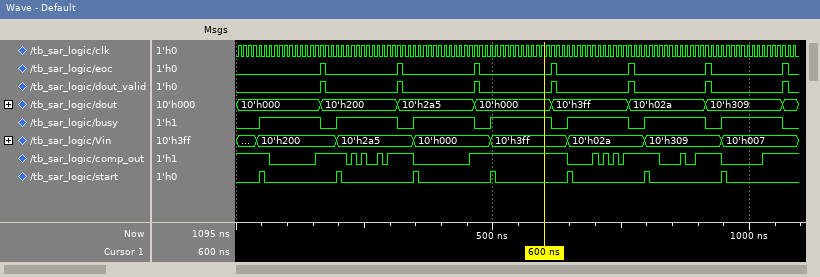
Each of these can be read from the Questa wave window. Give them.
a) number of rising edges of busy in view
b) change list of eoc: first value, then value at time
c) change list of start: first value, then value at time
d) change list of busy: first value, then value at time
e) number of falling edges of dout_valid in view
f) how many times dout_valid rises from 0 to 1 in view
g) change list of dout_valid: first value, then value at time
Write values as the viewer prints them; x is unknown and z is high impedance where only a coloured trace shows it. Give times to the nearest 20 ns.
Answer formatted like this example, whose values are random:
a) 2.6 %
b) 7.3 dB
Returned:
a) 7
b) 0, 1 at 160 ns, 0 at 180 ns, 1 at 320 ns, 0 at 320 ns, 1 at 460 ns, 0 at 480 ns, 1 at 620 ns, 0 at 620 ns, 1 at 760 ns, 0 at 780 ns, 1 at 920 ns, 0 at 920 ns, 1 at 1060 ns, 0 at 1080 ns
c) 0, 1 at 40 ns, 0 at 60 ns, 1 at 200 ns, 0 at 200 ns, 1 at 340 ns, 0 at 360 ns, 1 at 500 ns, 0 at 500 ns, 1 at 640 ns, 0 at 660 ns, 1 at 800 ns, 0 at 800 ns, 1 at 940 ns, 0 at 960 ns
d) 0, 1 at 40 ns, 0 at 160 ns, 1 at 200 ns, 0 at 320 ns, 1 at 340 ns, 0 at 460 ns, 1 at 500 ns, 0 at 620 ns, 1 at 640 ns, 0 at 760 ns, 1 at 800 ns, 0 at 920 ns, 1 at 940 ns, 0 at 1060 ns
e) 7
f) 7
g) 0, 1 at 160 ns, 0 at 180 ns, 1 at 320 ns, 0 at 320 ns, 1 at 460 ns, 0 at 480 ns, 1 at 620 ns, 0 at 620 ns, 1 at 760 ns, 0 at 780 ns, 1 at 920 ns, 0 at 920 ns, 1 at 1060 ns, 0 at 1080 ns
